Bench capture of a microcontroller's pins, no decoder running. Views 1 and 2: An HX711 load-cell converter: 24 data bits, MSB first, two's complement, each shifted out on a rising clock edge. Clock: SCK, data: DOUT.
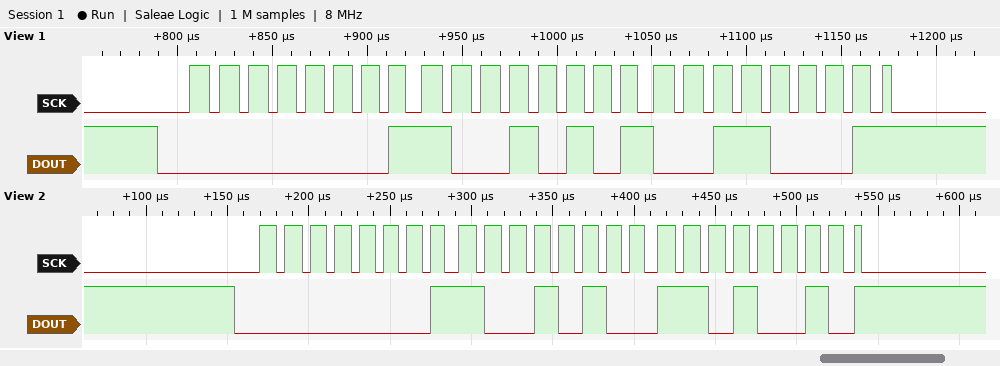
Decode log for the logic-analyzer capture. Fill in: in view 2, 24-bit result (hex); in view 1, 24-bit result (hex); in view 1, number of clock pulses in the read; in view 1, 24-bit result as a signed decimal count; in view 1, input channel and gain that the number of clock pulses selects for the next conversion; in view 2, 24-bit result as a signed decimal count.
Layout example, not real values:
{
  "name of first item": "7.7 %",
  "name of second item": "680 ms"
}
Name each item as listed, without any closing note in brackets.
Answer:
{
  "in view 2, 24-bit result": "0x0194D2",
  "in view 1, 24-bit result": "0x019531",
  "in view 1, number of clock pulses in the read": "25",
  "in view 1, 24-bit result as a signed decimal count": "103729",
  "in view 1, input channel and gain that the number of clock pulses selects for the next conversion": "channel A, gain 128",
  "in view 2, 24-bit result as a signed decimal count": "103634"
}
